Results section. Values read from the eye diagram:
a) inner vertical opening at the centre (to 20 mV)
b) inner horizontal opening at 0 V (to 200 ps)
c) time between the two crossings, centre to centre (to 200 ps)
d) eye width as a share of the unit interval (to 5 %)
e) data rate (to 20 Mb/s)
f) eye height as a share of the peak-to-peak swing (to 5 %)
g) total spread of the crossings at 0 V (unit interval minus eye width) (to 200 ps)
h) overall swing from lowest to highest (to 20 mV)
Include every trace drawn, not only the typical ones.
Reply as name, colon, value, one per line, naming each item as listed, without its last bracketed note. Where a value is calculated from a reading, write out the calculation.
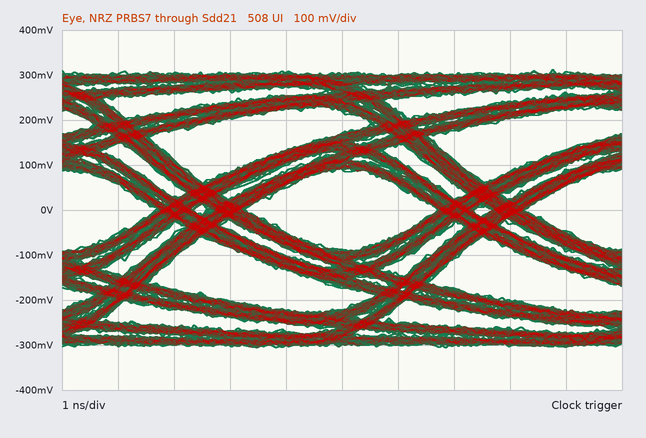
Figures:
inner vertical opening at the centre: 180 mV
inner horizontal opening at 0 V: 3.4 ns
time between the two crossings, centre to centre: 5.0 ns
eye width as a share of the unit interval: 3.4 ns / 5.0 ns ≈ 68.0 %, so 70 % to the nearest 5 %
data rate: 200 Mb/s
eye height as a share of the peak-to-peak swing: 180 mV / 620 mV ≈ 29.0 %, so 30 % to the nearest 5 %
total spread of the crossings at 0 V (unit interval minus eye width): 1.6 ns
overall swing from lowest to highest: 620 mV
